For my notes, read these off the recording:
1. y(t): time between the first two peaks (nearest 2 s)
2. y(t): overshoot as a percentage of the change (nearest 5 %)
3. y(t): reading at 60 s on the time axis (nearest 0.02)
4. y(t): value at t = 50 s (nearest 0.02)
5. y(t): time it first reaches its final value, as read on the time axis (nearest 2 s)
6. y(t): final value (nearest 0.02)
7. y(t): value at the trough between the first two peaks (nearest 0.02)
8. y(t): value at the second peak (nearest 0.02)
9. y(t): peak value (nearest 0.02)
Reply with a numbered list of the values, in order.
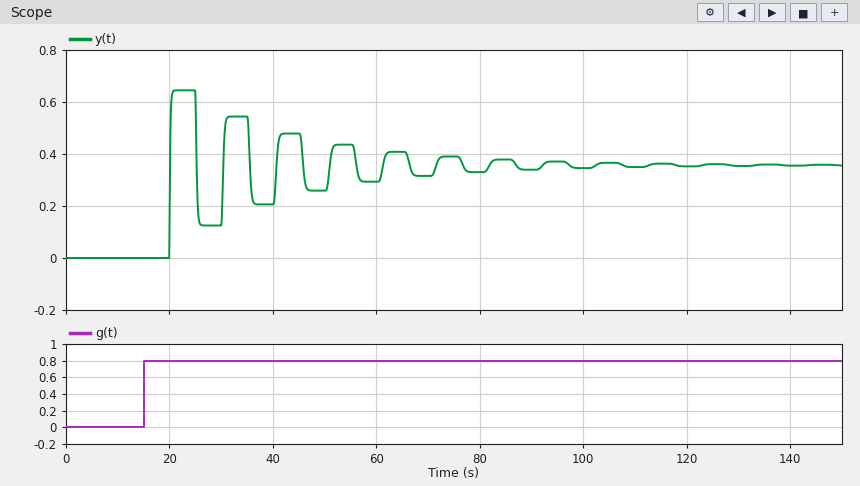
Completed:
1. 10 s
2. 80 %
3. 0.30
4. 0.26
5. 20 s
6. 0.36
7. 0.12
8. 0.54
9. 0.64
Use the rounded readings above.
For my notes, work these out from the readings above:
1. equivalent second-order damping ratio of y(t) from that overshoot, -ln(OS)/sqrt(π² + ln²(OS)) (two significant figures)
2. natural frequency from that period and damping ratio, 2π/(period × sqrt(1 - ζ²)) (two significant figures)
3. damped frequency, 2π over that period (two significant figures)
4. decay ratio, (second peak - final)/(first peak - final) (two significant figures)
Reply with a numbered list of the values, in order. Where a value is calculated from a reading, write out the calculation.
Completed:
1. ln(0.8) = -0.223; 0.223 / sqrt(9.870 + 0.050) = 0.071
2. 2π / (10 × sqrt(1 - 0.071²)) = 0.63 rad/s
3. 2π / 10 = 0.63 rad/s
4. (0.54 - 0.36) / (0.64 - 0.36) = 0.64
